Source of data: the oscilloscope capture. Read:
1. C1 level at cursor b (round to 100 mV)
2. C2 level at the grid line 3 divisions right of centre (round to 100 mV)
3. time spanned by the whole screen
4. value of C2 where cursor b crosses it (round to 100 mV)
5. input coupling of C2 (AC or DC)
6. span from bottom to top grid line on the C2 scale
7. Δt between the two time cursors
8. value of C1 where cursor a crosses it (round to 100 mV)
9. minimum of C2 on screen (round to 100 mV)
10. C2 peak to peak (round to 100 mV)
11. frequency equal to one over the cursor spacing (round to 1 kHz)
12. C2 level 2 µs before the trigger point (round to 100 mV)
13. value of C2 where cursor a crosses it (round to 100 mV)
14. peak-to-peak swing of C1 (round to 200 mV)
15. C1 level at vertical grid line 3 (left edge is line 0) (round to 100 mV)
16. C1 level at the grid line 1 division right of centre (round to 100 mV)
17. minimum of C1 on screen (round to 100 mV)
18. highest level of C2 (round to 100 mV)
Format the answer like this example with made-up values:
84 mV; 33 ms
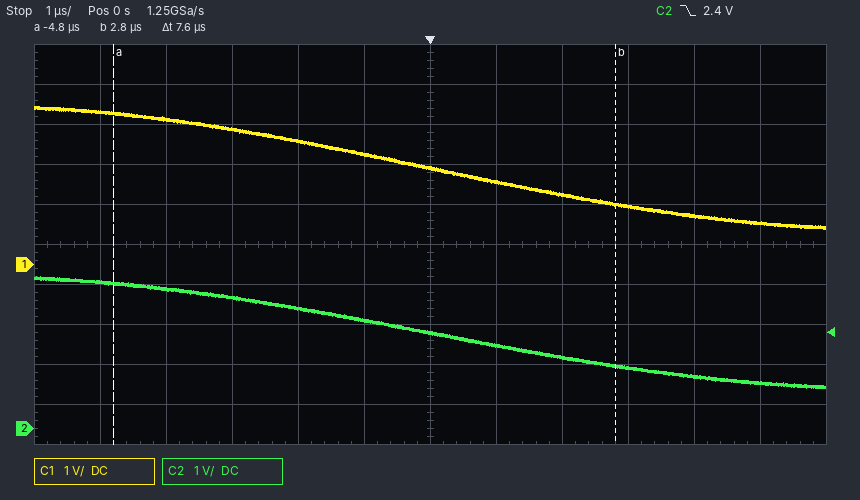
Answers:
1.5 V; 1.5 V; 12 µs; 1.6 V; DC; 10 V; 7.6 µs; 3.8 V; 1.0 V; 2.8 V; 132 kHz; 3.0 V; 3.6 V; 3.0 V; 3.4 V; 2.1 V; 900 mV; 3.8 V
